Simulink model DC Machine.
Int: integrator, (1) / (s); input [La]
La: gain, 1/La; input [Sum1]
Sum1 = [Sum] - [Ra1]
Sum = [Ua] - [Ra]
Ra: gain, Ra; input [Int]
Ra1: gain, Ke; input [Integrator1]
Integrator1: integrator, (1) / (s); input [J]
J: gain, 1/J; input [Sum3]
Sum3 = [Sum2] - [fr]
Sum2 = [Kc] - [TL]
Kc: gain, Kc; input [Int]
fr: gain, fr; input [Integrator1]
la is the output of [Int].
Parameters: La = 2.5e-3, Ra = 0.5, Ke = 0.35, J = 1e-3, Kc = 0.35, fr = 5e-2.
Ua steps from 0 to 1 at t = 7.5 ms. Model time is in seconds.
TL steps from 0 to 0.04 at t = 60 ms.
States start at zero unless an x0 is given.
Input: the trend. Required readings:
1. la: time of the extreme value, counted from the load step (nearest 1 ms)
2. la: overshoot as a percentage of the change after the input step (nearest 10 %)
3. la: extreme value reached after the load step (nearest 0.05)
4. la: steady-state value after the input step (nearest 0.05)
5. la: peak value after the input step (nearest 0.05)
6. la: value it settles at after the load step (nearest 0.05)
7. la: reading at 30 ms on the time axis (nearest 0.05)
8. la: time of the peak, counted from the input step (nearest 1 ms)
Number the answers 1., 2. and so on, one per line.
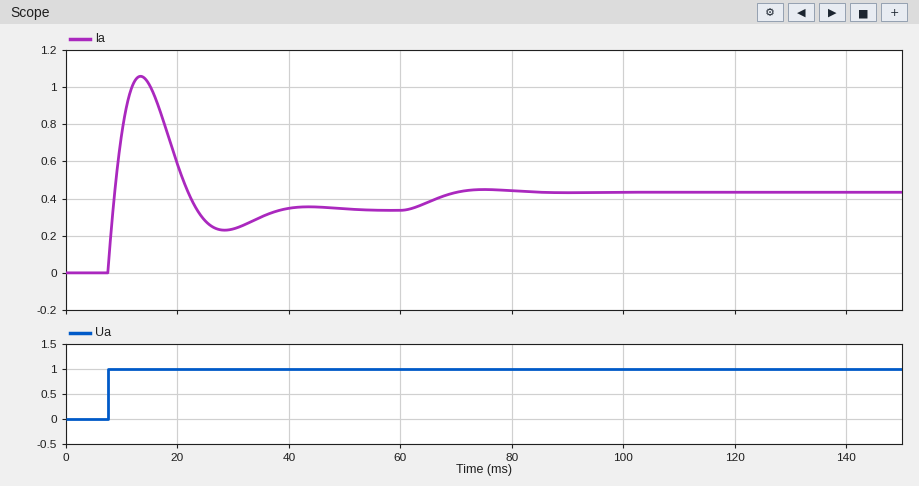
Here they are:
1. 15 ms
2. 210 %
3. 0.45
4. 0.35
5. 1.05
6. 0.45
7. 0.25
8. 6 ms
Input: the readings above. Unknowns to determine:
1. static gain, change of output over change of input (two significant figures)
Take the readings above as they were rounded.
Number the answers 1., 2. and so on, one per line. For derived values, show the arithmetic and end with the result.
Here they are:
1. (0.35 - 0) / (1 - 0) = 0.35
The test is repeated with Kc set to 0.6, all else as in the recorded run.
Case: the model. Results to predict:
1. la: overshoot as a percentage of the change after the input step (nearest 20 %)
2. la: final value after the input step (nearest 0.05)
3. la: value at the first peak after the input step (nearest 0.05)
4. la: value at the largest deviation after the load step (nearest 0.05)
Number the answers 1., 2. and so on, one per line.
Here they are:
1. 320 %
2. 0.20
3. 0.90
4. 0.30
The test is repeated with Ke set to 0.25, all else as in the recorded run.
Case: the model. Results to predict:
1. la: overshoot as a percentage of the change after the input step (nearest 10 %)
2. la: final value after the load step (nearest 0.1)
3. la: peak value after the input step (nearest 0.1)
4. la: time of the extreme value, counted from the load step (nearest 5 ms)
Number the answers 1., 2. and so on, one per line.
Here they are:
1. 160 %
2. 0.5
3. 1.2
4. 20 ms
